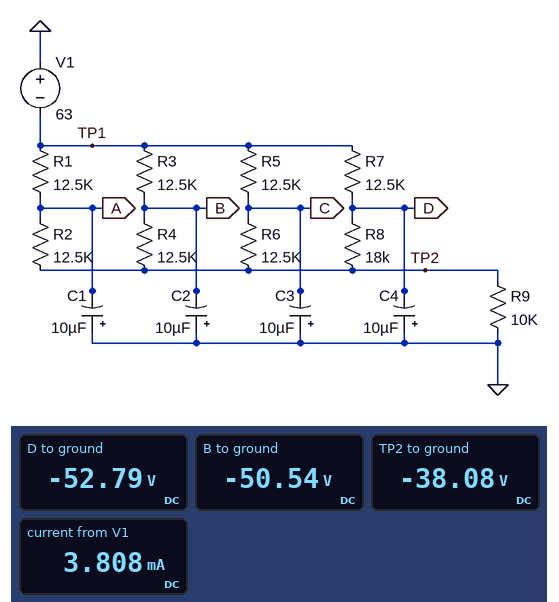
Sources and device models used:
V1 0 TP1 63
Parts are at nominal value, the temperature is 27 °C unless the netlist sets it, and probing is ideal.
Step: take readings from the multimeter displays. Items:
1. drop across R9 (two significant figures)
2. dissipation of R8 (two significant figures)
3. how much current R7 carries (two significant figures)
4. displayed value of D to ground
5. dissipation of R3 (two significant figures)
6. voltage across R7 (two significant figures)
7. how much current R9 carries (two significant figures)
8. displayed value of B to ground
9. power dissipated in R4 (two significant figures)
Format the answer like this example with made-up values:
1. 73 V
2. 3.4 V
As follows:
1. 38 V
2. 12 mW
3. 820 µA
4. -52.79 V
5. 12 mW
6. 10 V
7. 3.8 mA
8. -50.54 V
9. 12 mW
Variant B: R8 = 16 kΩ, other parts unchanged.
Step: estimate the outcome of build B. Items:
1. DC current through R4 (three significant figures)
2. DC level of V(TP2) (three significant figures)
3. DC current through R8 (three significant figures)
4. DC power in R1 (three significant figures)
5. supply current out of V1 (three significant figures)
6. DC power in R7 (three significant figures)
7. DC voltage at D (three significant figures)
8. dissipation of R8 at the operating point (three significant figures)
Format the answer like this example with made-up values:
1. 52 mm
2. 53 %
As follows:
1. 988 µA
2. -38.3 V
3. 867 µA
4. 12.2 mW
5. 3.83 mA
6. 9.39 mW
7. -52.2 V
8. 12.0 mW
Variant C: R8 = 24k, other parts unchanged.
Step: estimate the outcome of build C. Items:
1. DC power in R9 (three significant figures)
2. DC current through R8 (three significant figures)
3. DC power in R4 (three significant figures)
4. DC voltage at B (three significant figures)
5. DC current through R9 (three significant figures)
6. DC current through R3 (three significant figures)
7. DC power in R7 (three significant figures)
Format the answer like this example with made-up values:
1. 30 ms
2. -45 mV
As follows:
1. 141 mW
2. 698 µA
3. 13.0 mW
4. -50.3 V
5. 3.75 mA
6. 1.02 mA
7. 6.08 mW
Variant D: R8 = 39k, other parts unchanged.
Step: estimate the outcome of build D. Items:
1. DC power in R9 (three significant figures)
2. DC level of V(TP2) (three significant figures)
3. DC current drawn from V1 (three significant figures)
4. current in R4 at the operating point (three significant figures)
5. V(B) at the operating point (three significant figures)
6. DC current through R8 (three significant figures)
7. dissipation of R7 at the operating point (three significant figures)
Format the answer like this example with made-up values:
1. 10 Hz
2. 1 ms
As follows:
1. 135 mW
2. -36.7 V
3. 3.67 mA
4. 1.05 mA
5. -49.8 V
6. 511 µA
7. 3.26 mW
